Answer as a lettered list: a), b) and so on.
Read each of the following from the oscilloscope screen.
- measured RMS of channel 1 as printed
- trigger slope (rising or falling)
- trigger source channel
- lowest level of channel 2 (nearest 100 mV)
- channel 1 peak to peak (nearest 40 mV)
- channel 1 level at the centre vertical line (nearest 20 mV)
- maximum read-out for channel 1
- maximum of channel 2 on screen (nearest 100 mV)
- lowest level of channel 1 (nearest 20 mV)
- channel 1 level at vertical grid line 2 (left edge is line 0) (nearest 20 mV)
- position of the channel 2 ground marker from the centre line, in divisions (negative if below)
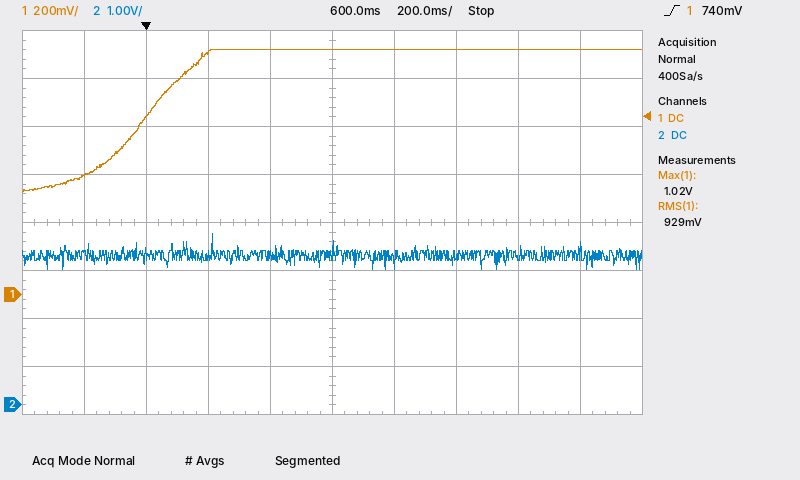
a) 929 mV
b) rising
c) channel 1
d) 2.8 V
e) 600 mV
f) 1.02 V
g) 1.02 V
h) 3.6 V
i) 420 mV
j) 740 mV
k) -3.8 div
